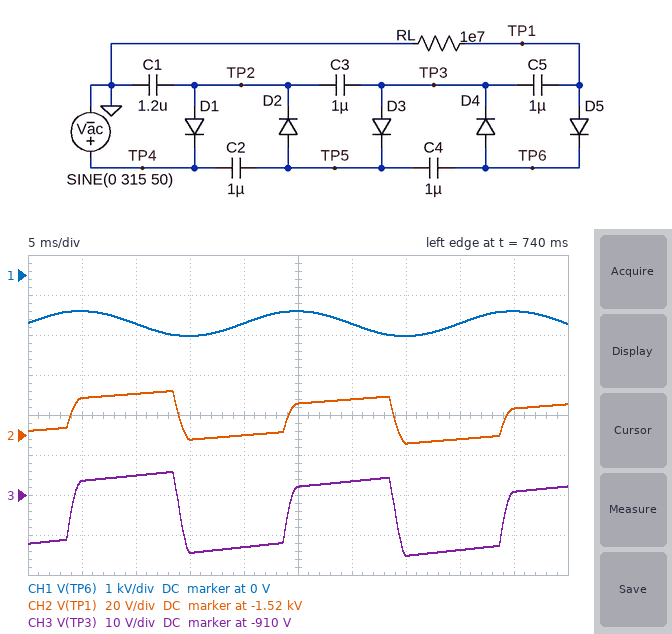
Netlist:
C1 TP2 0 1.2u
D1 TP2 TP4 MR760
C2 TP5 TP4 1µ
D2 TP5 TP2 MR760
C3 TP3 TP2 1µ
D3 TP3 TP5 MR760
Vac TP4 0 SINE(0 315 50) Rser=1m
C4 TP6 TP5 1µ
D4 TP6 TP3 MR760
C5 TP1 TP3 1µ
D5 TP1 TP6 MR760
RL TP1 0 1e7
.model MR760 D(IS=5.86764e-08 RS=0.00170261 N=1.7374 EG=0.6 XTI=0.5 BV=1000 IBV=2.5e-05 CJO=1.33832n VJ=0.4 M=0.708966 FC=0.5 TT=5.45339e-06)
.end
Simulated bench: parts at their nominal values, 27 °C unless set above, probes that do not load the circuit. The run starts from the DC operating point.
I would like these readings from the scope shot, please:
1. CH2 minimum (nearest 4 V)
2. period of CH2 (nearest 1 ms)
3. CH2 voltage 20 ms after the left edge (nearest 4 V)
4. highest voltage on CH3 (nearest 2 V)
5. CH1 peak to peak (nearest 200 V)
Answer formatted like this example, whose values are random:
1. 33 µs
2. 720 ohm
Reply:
1. -1.524 kV
2. 20 ms
3. -1.520 kV
4. -904 V
5. 600 V
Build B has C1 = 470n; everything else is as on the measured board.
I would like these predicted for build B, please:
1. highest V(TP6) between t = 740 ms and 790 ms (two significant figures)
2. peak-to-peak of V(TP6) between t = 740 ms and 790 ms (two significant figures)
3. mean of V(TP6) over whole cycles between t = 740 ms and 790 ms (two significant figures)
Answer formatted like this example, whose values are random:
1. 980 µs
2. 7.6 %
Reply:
1. -840 V
2. 610 V
3. -1.1 kV
